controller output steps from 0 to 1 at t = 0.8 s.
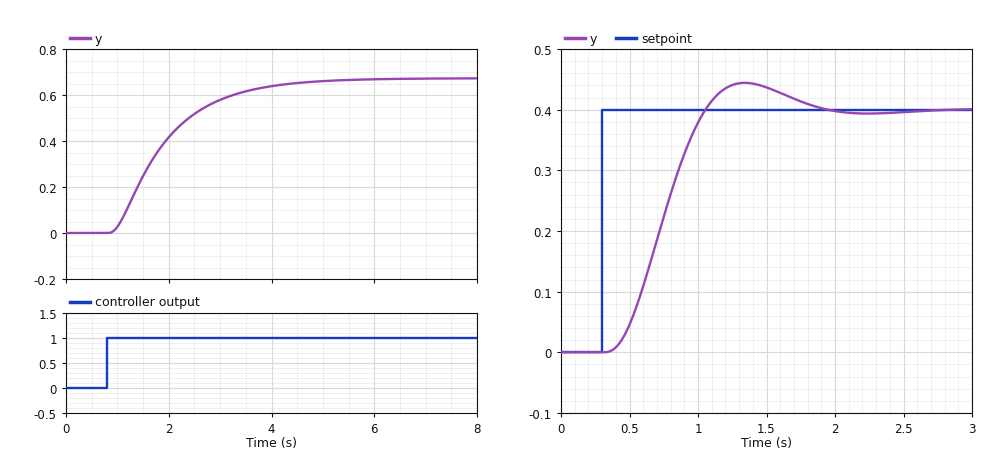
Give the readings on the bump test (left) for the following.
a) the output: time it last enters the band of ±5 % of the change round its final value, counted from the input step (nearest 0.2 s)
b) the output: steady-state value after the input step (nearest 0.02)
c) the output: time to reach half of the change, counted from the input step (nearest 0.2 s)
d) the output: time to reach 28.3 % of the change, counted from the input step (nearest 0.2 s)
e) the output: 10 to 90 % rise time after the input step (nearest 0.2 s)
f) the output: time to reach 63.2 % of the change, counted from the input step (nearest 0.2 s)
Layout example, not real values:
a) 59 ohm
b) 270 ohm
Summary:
a) 3.2 s
b) 0.68
c) 1.0 s
d) 0.6 s
e) 2.2 s
f) 1.2 s
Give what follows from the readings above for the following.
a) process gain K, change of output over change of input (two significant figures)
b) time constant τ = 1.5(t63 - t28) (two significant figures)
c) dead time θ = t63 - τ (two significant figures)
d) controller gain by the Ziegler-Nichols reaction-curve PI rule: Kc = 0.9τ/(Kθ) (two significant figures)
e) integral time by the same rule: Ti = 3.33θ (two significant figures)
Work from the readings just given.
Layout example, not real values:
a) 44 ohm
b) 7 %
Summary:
a) 0.68
b) 0.90 s
c) 0.30 s
d) 4.0
e) 1.00 s
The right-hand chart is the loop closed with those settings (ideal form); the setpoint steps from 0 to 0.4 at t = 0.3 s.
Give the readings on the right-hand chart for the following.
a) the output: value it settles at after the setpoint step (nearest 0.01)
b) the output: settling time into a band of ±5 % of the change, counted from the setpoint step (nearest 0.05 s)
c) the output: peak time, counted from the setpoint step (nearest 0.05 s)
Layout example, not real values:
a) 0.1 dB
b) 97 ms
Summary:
a) 0.40
b) 1.40 s
c) 1.05 s
